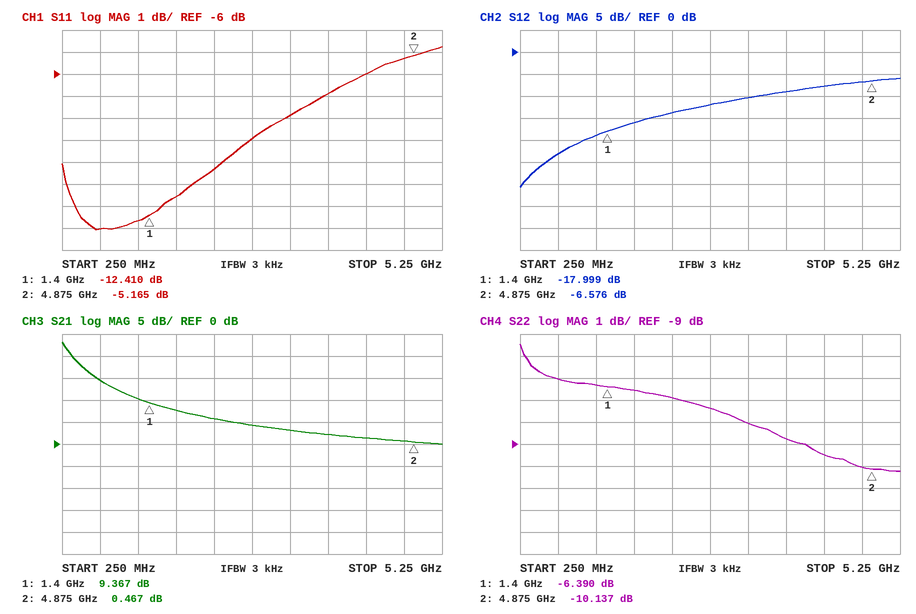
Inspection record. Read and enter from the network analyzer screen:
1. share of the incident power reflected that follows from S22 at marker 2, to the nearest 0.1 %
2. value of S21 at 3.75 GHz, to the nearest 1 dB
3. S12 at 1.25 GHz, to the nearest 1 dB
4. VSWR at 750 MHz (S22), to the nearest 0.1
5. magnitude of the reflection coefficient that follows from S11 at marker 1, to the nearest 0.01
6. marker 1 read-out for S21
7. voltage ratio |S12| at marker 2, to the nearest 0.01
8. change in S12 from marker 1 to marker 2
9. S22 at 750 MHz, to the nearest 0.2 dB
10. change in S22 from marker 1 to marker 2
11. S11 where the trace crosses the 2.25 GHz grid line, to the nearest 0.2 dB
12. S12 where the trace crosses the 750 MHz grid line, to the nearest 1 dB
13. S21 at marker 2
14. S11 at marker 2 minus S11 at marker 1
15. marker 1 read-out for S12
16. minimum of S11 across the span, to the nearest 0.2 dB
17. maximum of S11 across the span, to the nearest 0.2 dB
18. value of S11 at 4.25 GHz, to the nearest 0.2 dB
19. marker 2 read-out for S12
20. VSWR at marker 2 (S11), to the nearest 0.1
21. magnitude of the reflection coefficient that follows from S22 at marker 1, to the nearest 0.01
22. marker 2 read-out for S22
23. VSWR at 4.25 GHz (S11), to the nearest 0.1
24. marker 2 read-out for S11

9.7 %
2 dB
-19 dB
3.0
0.24
9.367 dB
0.47
11.423 dB
-6.0 dB
-3.747 dB
-10.4 dB
-23 dB
0.467 dB
7.245 dB
-17.999 dB
-13.0 dB
-4.8 dB
-6.0 dB
-6.576 dB
3.5
0.48
-10.137 dB
3.0
-5.165 dB
